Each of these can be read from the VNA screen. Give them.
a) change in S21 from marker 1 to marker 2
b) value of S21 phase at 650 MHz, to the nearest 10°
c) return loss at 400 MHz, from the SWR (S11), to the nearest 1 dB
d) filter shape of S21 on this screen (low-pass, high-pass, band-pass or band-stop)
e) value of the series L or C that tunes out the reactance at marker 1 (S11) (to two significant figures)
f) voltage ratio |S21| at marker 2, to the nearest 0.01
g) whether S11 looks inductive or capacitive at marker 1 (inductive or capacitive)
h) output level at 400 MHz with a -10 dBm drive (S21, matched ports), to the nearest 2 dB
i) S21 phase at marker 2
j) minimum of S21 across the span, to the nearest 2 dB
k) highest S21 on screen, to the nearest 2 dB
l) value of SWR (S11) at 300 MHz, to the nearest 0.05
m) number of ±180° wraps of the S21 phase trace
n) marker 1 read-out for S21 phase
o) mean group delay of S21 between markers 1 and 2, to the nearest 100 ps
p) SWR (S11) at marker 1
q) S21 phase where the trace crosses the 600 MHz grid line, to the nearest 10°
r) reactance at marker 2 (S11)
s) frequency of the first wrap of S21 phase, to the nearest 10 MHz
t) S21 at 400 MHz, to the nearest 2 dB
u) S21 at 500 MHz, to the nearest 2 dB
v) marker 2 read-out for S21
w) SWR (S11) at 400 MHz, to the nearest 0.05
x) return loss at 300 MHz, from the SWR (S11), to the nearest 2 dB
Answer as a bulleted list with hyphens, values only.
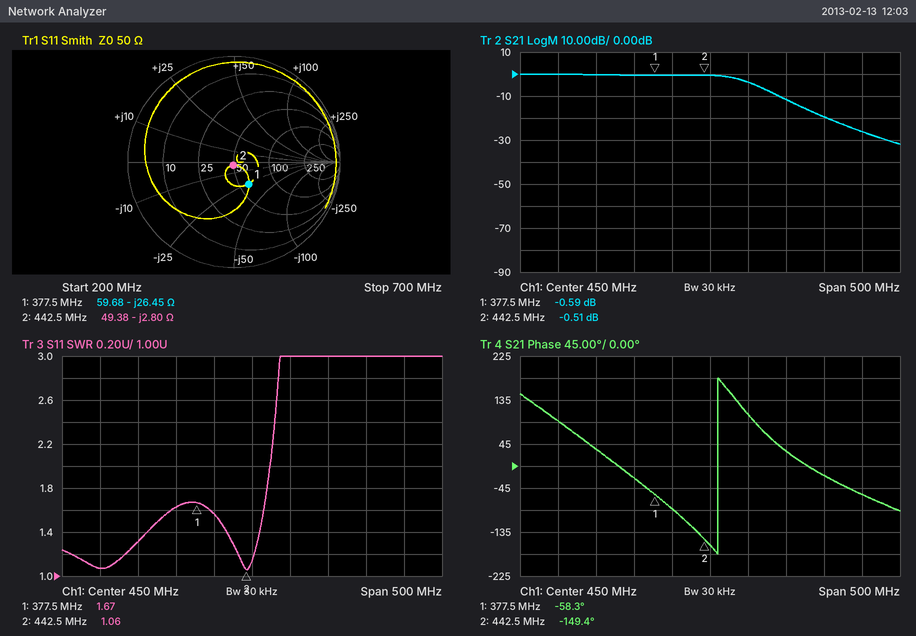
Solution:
- 0.08 dB
- -60°
- 13 dB
- low-pass
- 11 nH
- 0.94
- capacitive
- -10 dBm
- -149.4°
- -32 dB
- 0 dB
- 1.30
- 1
- -58.3°
- 3.9 ns
- 1.67
- -20°
- -2.80 Ω
- 460 MHz
- 0 dB
- -4 dB
- -0.51 dB
- 1.55
- 18 dB
